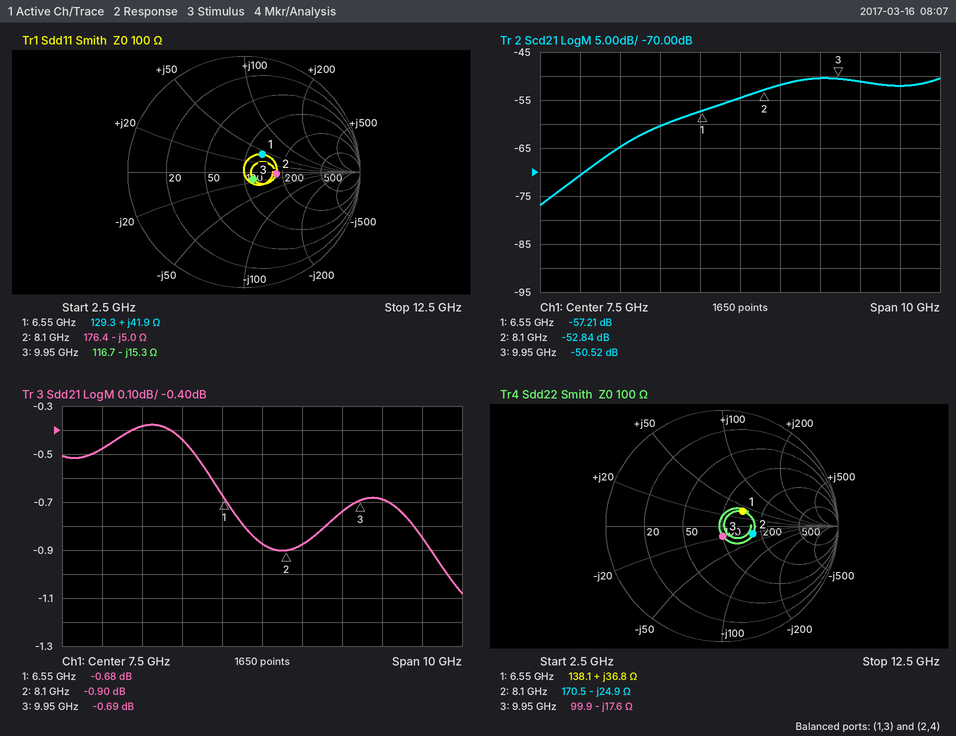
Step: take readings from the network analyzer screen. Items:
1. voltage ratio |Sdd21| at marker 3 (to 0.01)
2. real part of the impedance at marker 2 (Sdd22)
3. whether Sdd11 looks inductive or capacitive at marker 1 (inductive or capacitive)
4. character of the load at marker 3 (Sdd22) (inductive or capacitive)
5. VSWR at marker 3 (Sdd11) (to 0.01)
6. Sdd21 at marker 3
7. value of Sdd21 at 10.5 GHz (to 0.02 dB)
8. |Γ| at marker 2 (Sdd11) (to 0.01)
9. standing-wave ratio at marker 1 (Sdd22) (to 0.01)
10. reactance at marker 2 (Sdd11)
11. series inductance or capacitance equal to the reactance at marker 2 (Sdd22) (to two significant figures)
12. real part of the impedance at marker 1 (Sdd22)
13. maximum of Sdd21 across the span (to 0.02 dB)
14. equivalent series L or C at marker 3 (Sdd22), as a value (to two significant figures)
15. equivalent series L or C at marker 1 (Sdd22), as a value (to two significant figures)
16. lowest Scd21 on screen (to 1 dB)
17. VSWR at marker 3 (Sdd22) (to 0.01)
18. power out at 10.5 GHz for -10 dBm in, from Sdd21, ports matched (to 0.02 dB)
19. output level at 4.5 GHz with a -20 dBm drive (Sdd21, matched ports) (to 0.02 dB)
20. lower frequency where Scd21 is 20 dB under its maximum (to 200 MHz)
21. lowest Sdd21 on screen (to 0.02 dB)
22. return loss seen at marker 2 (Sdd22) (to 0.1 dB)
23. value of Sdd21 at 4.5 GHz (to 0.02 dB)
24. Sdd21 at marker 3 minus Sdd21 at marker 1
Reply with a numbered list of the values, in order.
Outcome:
1. 0.92
2. 170.5 Ω
3. inductive
4. capacitive
5. 1.23
6. -0.69 dB
7. -0.68 dB
8. 0.28
9. 1.56
10. -5.0 Ω
11. 790 fF
12. 138.1 Ω
13. -0.38 dB
14. 910 fF
15. 890 pH
16. -77 dB
17. 1.19
18. -10.68 dBm
19. -20.38 dBm
20. 3.6 GHz
21. -1.08 dB
22. 11.2 dB
23. -0.38 dB
24. -0.01 dB
